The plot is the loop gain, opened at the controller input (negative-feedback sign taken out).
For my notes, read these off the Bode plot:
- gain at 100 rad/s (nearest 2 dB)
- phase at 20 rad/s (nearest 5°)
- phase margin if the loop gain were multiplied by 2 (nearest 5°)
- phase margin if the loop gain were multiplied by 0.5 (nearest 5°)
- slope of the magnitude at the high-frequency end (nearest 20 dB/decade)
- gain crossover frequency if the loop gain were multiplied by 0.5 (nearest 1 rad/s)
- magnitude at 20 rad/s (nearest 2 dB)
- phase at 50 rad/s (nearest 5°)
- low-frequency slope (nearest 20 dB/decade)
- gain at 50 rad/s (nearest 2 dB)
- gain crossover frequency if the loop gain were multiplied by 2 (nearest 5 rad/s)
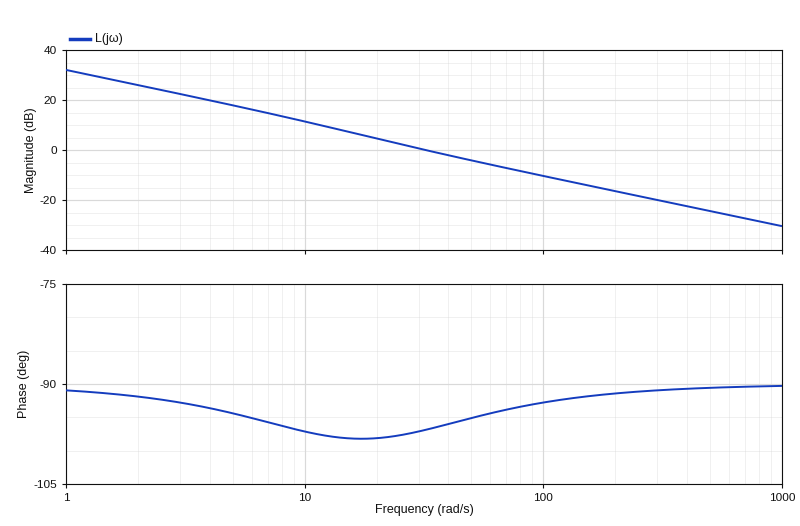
-10 dB
-100°
85°
80°
-20 dB/decade
17 rad/s
4 dB
-95°
-20 dB/decade
-4 dB
60 rad/s
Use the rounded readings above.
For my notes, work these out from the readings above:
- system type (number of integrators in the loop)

1
